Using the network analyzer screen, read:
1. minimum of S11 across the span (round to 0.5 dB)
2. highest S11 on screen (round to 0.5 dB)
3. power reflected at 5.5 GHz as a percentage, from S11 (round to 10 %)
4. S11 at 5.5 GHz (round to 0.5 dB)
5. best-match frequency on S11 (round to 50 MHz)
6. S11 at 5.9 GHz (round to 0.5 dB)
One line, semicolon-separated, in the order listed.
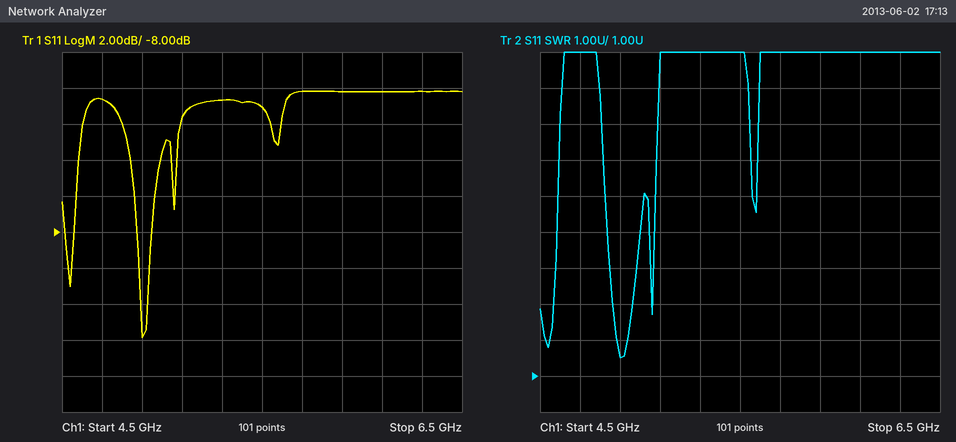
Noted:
-14.0 dB; 0.0 dB; 80 %; -1.0 dB; 4.90 GHz; 0.0 dB
